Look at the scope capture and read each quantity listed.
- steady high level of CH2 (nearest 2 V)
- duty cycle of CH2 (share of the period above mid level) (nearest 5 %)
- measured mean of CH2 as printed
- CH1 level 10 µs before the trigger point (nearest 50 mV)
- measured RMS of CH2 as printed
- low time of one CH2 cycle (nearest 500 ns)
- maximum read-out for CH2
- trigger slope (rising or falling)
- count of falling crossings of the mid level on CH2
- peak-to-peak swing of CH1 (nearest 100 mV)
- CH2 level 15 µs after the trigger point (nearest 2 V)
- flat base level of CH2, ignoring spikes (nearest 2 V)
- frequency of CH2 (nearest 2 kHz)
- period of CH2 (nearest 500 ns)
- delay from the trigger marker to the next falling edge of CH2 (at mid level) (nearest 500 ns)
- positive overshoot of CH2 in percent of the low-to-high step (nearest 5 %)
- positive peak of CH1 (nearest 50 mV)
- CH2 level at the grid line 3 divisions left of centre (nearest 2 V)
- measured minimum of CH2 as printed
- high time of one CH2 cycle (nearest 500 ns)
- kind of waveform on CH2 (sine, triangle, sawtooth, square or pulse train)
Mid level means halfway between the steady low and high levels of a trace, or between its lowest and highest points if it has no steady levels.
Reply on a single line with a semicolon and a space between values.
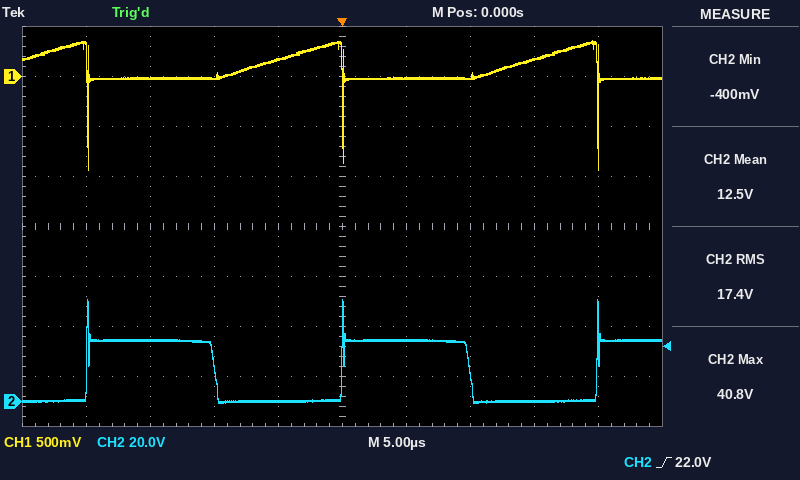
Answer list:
24 V; 50 %; 12.5 V; 0 mV; 17.4 V; 10.0 µs; 40.8 V; rising; 2; 1.30 V; 0 V; 0 V; 50 kHz; 20.0 µs; 10.0 µs; 65 %; 350 mV; 24 V; -400 mV; 10.0 µs; square
